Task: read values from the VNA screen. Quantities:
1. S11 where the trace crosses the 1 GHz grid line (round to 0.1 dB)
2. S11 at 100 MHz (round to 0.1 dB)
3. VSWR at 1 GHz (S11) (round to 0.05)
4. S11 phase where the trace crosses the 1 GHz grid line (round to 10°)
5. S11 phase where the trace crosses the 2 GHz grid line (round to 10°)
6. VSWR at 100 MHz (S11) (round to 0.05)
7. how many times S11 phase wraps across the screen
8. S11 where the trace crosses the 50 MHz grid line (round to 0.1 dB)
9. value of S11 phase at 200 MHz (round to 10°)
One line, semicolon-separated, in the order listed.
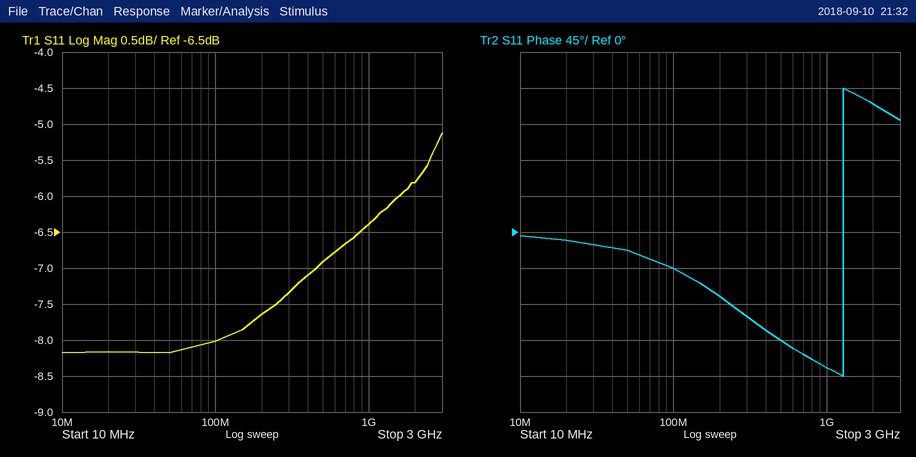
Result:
-6.4 dB; -8.0 dB; 2.85; -170°; 160°; 2.30; 1; -8.2 dB; -80°
